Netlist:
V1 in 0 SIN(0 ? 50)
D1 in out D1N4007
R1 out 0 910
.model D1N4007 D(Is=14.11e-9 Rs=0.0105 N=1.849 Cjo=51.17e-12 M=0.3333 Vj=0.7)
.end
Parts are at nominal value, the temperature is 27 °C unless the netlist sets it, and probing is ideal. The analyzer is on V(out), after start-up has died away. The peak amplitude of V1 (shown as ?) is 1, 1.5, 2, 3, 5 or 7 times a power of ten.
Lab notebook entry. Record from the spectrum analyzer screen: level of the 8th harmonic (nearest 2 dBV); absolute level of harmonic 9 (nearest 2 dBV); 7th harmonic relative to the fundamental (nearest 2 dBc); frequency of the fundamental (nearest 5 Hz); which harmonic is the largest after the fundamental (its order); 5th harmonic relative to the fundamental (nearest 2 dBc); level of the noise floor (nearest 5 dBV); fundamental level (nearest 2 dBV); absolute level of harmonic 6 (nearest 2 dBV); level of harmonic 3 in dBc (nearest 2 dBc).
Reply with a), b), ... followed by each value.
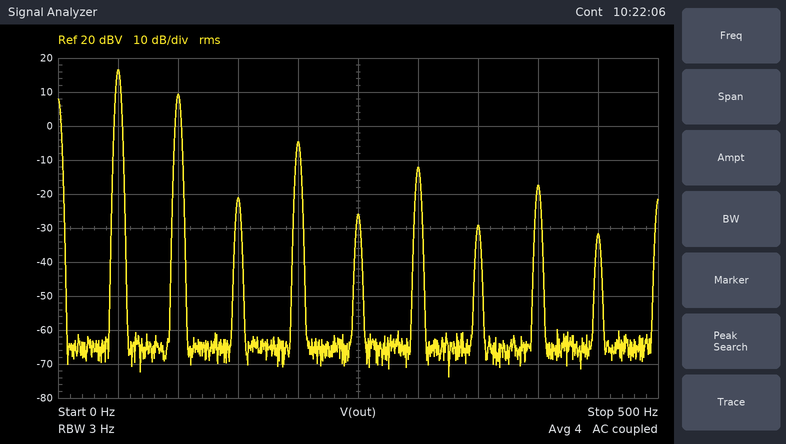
a) -18 dBV
b) -32 dBV
c) -46 dBc
d) 50 Hz
e) 2
f) -42 dBc
g) -65 dBV
h) 16 dBV
i) -12 dBV
j) -38 dBc
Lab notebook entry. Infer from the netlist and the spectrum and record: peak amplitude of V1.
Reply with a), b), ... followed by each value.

a) 20 V
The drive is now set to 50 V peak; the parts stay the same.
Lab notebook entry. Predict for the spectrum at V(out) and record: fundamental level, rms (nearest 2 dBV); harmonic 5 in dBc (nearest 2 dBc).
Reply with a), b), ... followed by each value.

a) 24 dBV
b) -50 dBc
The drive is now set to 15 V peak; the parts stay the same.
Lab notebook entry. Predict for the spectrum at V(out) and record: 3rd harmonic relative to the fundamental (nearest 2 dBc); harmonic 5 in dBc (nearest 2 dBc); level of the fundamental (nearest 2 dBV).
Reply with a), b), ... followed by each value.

a) -36 dBc
b) -40 dBc
c) 14 dBV
